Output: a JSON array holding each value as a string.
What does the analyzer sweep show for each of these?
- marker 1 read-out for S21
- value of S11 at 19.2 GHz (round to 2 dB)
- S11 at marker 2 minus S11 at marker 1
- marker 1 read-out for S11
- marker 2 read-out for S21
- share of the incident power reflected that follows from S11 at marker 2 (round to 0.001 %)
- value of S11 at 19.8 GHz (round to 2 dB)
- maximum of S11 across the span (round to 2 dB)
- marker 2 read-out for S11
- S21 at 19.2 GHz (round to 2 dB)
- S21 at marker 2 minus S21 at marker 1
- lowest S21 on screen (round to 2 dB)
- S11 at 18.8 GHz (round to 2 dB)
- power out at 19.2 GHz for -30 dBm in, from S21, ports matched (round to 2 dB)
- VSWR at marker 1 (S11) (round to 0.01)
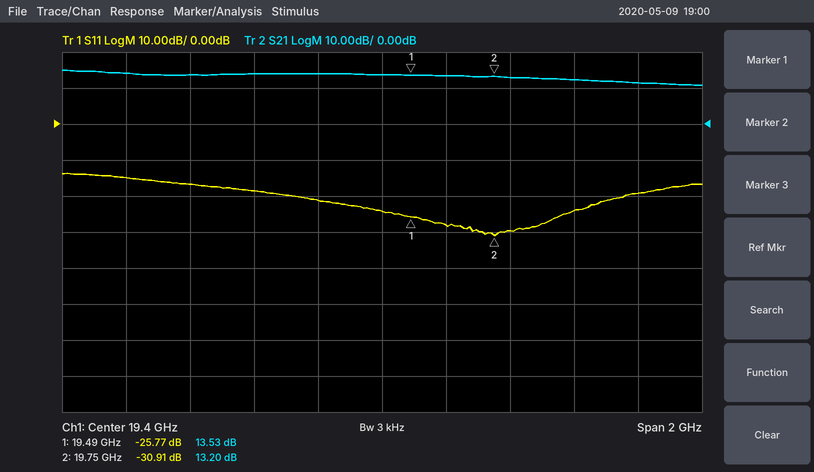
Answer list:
["13.53 dB", "-22 dB", "-5.14 dB", "-25.77 dB", "13.20 dB", "0.081 %", "-30 dB", "-14 dB", "-30.91 dB", "14 dB", "-0.33 dB", "10 dB", "-16 dB", "-16 dBm", "1.11"]
